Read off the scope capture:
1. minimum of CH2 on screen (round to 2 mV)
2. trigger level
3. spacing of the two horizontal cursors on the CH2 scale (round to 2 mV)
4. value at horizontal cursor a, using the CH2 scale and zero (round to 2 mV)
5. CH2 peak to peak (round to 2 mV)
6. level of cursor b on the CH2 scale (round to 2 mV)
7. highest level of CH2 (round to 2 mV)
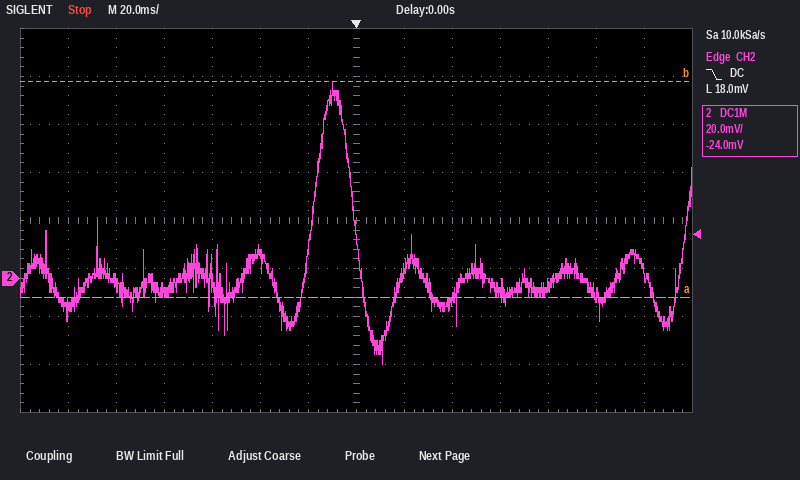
-36 mV
18.0 mV
90 mV
-8 mV
118 mV
82 mV
82 mV
